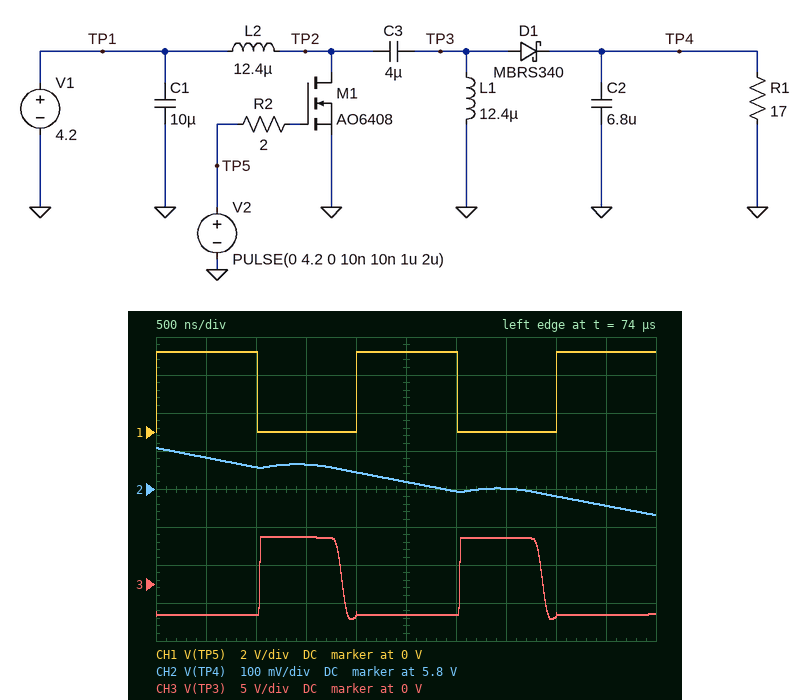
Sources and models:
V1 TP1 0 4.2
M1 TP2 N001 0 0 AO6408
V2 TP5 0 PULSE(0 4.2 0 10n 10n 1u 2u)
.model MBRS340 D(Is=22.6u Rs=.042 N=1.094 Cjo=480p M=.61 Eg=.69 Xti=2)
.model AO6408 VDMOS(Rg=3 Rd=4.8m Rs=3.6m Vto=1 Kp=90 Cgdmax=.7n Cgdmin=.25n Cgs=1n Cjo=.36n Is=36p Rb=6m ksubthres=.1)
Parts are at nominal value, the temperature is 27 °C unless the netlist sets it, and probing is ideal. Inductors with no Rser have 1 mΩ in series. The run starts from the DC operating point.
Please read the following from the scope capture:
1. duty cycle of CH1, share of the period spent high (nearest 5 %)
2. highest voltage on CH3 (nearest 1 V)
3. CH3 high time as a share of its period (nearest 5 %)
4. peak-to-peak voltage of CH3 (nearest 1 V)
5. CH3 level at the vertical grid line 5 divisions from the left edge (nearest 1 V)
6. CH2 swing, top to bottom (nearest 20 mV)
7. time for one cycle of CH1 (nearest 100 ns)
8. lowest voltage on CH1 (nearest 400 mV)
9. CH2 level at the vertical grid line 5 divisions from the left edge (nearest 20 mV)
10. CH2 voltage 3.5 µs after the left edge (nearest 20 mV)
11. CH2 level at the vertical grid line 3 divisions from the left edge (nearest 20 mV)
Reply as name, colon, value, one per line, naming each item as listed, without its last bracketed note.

duty cycle of CH1, share of the period spent high: 50 %
highest voltage on CH3: 6 V
CH3 high time as a share of its period: 40 %
peak-to-peak voltage of CH3: 11 V
CH3 level at the vertical grid line 5 divisions from the left edge: -4 V
CH2 swing, top to bottom: 180 mV
time for one cycle of CH1: 2.0 µs
lowest voltage on CH1: 0 V
CH2 level at the vertical grid line 5 divisions from the left edge: 5.82 V
CH2 voltage 3.5 µs after the left edge: 5.80 V
CH2 level at the vertical grid line 3 divisions from the left edge: 5.86 V
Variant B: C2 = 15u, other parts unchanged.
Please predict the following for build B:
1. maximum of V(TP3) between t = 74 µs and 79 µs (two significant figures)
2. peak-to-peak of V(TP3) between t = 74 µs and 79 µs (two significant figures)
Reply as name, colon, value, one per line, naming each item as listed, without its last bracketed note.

maximum of V(TP3) between t = 74 µs and 79 µs: 7.2 V
peak-to-peak of V(TP3) between t = 74 µs and 79 µs: 12 V
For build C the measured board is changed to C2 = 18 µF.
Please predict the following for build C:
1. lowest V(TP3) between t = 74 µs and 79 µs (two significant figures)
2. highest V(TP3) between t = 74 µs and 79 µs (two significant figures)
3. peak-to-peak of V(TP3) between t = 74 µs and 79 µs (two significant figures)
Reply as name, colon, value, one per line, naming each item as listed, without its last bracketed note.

lowest V(TP3) between t = 74 µs and 79 µs: -4.8 V
highest V(TP3) between t = 74 µs and 79 µs: 7.3 V
peak-to-peak of V(TP3) between t = 74 µs and 79 µs: 12 V
